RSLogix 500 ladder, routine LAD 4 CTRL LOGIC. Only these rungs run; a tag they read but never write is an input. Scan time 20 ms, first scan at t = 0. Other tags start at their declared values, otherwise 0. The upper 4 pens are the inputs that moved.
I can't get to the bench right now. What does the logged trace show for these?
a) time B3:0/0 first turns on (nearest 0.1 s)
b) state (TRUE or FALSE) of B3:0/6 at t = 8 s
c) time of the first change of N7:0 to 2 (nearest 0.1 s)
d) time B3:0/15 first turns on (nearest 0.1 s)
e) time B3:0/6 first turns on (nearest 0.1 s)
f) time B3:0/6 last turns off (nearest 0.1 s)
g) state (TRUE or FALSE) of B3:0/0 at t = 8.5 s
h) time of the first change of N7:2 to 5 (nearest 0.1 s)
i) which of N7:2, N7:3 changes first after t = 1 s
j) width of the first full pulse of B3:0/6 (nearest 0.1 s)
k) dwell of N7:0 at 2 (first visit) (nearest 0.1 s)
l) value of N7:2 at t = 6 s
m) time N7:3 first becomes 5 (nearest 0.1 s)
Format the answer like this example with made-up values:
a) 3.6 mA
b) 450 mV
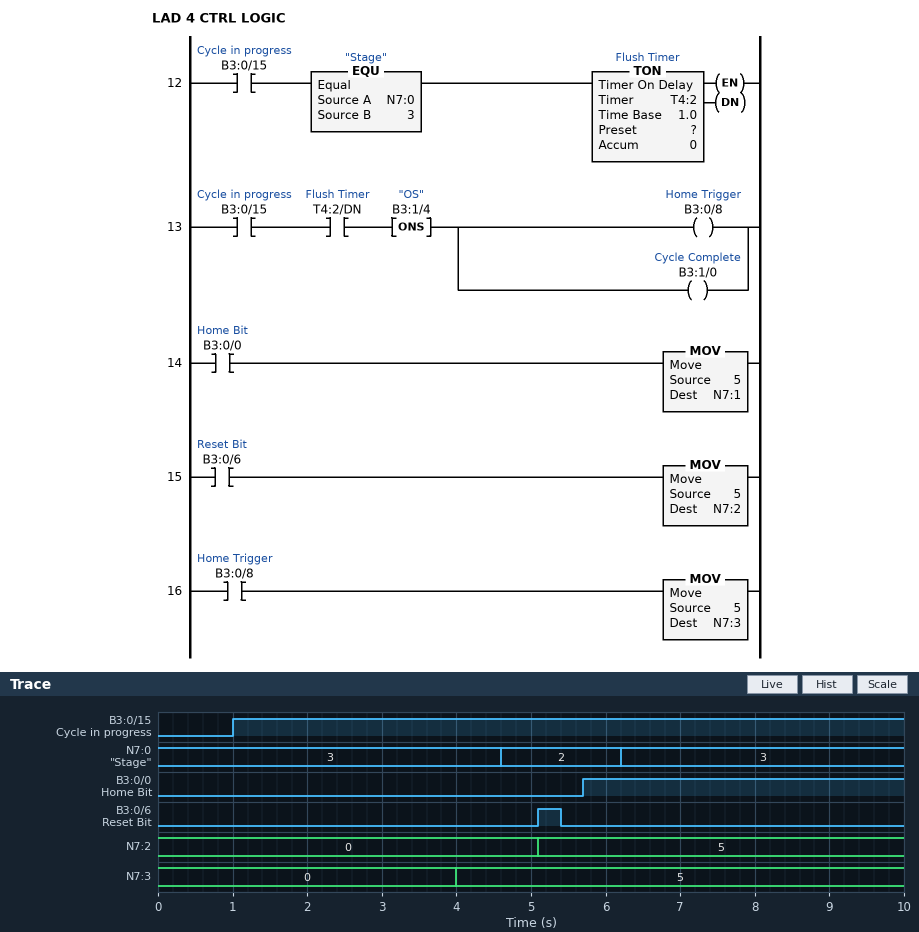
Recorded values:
a) 5.7 s
b) FALSE
c) 4.6 s
d) 1.0 s
e) 5.1 s
f) 5.4 s
g) TRUE
h) 5.1 s
i) N7:3
j) 0.3 s
k) 1.6 s
l) 5
m) 4.0 s
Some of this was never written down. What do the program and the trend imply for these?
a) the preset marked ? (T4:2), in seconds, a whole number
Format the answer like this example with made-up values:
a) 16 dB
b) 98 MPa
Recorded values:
a) 3 s
